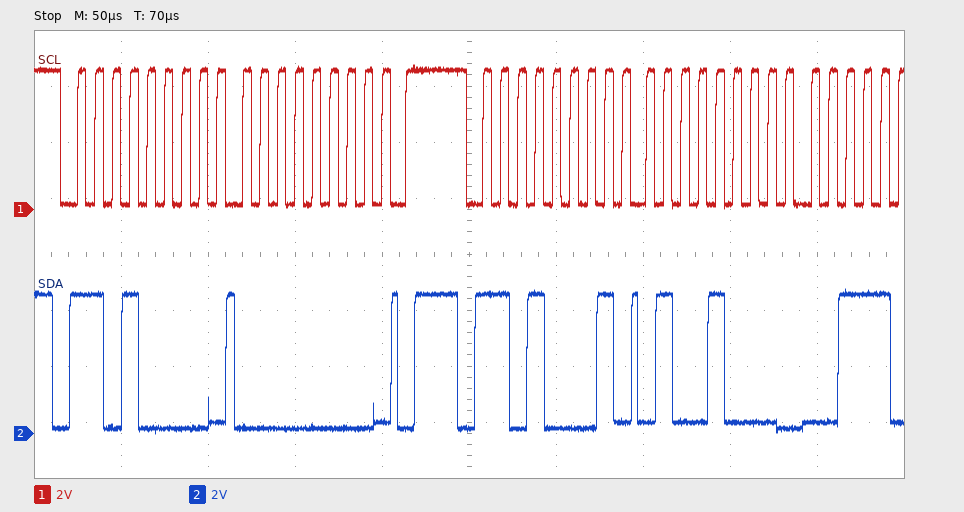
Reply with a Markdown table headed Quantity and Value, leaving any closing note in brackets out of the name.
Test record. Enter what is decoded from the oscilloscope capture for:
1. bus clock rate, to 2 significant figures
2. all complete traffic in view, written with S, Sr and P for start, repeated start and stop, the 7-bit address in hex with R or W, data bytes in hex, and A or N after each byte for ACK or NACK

| Quantity | Value |
|---|---|
| bus clock rate, to 2 significant figures | 100 kHz |
| all complete traffic in view, written with S, Sr and P for start, repeated start and stop, the 7-bit address in hex with R or W, data bytes in hex, and A or N after each byte for ACK or NACK | S 68W A 00 A P S 68R A 48 A |
